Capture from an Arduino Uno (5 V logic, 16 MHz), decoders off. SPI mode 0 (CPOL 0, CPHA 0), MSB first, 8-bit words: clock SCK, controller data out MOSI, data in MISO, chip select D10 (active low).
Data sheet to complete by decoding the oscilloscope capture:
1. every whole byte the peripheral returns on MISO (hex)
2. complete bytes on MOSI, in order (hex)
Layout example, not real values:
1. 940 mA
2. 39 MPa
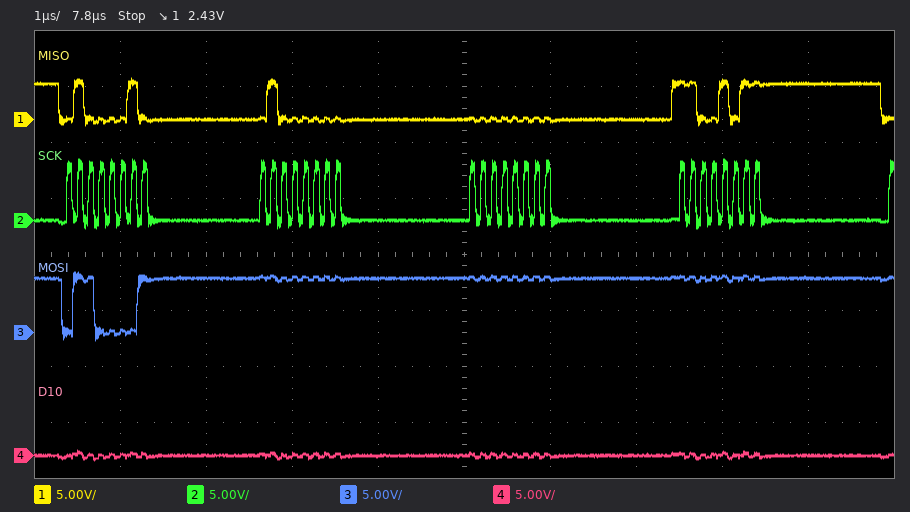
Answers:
1. 0x42 0x40 0x00 0xCB
2. 0x61 0xFF 0xFF 0xFF
